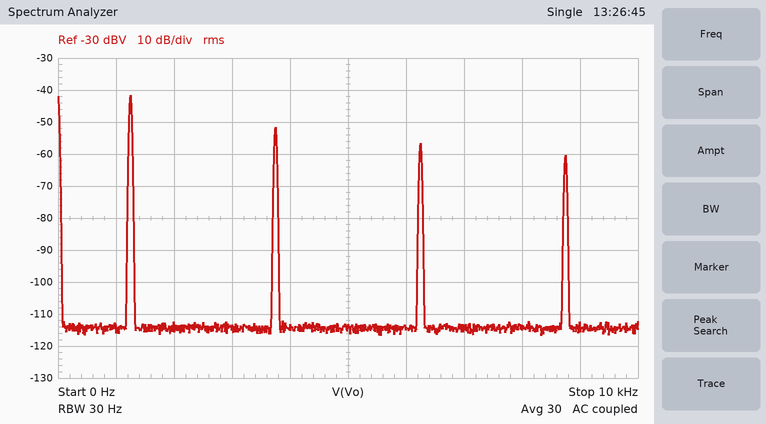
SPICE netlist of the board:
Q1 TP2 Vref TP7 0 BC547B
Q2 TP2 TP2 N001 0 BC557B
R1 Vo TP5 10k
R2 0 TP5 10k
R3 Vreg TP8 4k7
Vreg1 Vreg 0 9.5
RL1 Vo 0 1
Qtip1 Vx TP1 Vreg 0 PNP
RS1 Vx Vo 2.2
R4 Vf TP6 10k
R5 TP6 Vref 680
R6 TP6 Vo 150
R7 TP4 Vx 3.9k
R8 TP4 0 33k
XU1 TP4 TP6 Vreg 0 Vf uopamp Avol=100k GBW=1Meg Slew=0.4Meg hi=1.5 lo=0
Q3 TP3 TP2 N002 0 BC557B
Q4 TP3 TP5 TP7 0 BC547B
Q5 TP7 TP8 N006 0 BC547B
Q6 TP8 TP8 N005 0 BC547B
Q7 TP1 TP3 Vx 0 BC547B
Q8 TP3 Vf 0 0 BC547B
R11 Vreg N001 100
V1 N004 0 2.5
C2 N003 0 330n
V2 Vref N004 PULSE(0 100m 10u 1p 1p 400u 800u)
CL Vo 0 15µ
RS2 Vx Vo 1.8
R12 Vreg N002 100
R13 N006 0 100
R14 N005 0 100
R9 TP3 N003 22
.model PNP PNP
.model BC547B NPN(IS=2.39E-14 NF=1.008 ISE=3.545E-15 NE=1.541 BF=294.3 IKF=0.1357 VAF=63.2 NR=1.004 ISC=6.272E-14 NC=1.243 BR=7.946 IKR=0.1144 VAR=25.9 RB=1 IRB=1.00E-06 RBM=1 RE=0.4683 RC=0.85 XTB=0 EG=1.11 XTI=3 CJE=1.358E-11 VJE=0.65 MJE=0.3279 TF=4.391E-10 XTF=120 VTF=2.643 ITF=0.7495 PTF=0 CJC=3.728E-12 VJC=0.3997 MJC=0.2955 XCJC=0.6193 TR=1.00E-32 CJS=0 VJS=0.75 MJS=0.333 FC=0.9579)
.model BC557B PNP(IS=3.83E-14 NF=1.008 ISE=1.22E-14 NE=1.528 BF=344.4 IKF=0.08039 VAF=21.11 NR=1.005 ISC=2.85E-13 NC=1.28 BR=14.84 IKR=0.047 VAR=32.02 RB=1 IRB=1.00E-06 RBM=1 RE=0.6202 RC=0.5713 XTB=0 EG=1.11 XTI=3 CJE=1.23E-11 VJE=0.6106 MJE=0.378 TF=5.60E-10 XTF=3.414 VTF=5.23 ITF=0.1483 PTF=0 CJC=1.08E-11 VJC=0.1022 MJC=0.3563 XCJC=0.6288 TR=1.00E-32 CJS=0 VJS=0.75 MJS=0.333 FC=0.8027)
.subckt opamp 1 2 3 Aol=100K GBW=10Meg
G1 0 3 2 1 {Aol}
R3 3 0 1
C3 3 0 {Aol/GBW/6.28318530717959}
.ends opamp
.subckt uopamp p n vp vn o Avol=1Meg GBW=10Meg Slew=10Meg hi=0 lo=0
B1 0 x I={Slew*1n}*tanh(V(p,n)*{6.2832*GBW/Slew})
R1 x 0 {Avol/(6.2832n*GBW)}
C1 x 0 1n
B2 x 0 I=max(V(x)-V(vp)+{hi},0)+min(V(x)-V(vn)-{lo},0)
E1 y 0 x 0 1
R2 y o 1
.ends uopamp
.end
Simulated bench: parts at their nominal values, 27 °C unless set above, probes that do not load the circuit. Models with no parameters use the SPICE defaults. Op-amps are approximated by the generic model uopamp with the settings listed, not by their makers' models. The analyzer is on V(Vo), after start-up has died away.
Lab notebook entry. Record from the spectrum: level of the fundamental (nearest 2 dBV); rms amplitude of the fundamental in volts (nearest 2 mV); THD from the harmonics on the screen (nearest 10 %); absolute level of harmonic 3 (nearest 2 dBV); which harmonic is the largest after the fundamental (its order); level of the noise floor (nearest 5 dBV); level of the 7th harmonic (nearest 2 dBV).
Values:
-42 dBV
8 mV
40 %
-52 dBV
3
-115 dBV
-60 dBV
